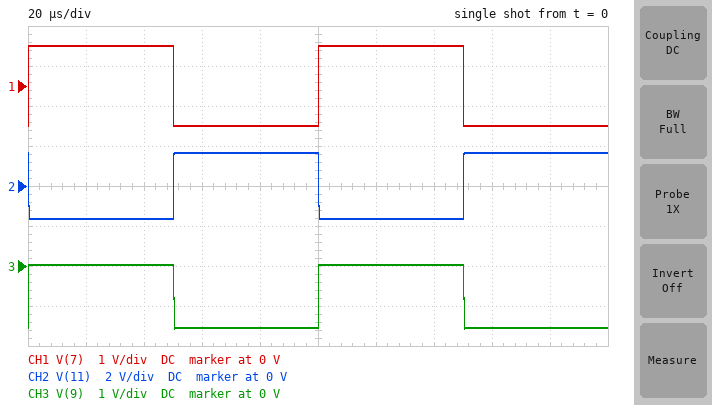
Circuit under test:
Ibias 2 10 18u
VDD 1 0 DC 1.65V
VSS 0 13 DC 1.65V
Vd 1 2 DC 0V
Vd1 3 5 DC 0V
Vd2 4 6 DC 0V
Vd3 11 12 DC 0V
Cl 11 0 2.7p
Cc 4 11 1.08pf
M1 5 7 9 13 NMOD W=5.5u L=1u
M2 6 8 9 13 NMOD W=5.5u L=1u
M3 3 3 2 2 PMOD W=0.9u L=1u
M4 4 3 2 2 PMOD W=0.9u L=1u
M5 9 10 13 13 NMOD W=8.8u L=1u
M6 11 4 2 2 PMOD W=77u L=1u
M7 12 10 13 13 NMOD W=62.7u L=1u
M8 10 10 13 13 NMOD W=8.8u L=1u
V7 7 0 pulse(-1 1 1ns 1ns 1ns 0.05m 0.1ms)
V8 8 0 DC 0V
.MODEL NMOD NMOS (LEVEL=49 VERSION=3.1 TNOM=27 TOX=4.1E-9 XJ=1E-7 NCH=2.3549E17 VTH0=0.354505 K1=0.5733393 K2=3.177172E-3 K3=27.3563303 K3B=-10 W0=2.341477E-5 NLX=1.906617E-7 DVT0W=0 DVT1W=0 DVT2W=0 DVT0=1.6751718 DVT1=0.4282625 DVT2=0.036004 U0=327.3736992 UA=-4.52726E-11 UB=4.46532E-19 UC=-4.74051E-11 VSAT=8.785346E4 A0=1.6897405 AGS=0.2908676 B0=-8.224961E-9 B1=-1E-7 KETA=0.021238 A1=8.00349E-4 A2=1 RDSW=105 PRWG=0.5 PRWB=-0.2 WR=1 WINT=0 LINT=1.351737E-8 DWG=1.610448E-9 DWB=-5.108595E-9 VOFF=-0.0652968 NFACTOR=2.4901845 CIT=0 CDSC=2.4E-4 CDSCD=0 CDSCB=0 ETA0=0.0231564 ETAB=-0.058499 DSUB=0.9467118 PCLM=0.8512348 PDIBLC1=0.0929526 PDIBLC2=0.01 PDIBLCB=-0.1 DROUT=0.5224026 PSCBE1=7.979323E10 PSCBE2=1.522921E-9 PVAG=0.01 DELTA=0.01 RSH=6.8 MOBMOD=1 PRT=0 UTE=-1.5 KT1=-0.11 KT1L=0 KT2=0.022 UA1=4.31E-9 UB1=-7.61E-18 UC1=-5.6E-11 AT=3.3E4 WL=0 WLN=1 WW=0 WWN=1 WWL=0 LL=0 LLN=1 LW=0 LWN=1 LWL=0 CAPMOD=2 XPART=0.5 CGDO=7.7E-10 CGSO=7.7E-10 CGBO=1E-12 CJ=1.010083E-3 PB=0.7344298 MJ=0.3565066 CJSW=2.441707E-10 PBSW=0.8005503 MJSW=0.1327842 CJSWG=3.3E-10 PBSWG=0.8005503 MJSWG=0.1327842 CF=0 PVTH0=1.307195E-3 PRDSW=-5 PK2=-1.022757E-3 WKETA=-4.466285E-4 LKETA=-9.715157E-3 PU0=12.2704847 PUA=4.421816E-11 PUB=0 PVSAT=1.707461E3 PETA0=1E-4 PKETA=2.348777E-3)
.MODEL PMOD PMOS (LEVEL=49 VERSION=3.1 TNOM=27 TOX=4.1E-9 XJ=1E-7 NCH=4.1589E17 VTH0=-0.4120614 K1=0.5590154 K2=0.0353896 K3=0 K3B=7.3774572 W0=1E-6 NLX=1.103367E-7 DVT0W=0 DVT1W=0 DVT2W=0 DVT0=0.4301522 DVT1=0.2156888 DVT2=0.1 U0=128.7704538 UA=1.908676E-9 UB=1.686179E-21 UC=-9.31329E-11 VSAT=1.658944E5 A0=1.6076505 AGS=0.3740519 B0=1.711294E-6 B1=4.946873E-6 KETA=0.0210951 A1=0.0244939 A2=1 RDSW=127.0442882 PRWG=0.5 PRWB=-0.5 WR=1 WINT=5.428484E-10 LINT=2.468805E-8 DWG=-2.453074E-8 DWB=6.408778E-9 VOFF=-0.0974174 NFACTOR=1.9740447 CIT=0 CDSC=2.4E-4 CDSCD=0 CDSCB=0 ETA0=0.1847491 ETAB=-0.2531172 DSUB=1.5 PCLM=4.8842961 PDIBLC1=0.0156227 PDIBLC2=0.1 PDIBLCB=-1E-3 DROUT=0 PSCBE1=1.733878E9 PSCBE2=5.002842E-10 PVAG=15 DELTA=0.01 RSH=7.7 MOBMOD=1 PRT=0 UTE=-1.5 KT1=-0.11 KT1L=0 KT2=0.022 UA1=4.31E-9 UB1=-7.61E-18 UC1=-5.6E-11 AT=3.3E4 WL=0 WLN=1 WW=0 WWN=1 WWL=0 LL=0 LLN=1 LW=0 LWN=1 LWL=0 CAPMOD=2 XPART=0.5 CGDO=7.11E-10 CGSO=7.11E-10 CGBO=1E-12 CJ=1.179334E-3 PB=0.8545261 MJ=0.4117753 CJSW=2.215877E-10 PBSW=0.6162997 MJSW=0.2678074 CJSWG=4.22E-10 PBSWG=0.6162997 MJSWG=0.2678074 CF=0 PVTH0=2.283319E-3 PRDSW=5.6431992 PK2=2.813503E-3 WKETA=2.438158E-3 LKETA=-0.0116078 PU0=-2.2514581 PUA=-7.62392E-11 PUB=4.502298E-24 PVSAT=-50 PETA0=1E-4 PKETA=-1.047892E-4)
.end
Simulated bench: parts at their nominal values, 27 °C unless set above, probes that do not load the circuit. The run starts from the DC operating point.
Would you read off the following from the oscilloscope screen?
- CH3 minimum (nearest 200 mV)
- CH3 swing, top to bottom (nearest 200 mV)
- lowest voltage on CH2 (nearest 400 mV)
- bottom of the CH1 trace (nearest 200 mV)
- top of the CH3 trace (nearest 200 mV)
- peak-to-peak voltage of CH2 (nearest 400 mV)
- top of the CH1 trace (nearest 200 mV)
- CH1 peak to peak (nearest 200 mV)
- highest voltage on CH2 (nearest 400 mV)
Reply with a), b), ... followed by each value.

a) -1.6 V
b) 1.6 V
c) -1.6 V
d) -1.0 V
e) 0 V
f) 3.2 V
g) 1.0 V
h) 2.0 V
i) 1.6 V
